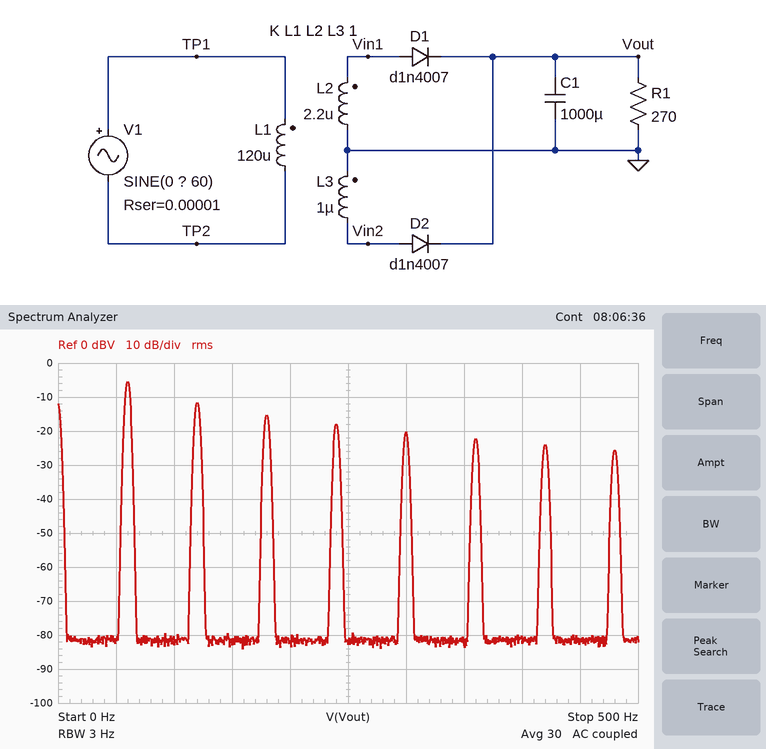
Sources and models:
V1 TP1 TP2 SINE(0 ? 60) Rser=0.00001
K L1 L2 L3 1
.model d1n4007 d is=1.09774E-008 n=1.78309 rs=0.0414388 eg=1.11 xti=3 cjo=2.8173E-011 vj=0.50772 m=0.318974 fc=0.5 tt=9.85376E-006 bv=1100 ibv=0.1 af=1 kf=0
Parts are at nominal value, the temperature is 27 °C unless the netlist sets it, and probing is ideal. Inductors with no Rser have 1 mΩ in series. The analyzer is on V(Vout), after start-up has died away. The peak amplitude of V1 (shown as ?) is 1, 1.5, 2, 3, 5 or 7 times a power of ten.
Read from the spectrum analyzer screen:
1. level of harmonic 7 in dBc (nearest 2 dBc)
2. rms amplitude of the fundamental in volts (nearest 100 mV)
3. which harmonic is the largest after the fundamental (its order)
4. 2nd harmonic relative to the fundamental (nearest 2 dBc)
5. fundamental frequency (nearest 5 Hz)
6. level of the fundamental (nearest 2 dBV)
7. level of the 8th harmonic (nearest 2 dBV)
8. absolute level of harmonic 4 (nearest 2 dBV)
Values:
-18 dBc
500 mV
2
-6 dBc
60 Hz
-6 dBV
-26 dBV
-18 dBV
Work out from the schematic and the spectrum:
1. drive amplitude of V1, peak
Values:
300 V
